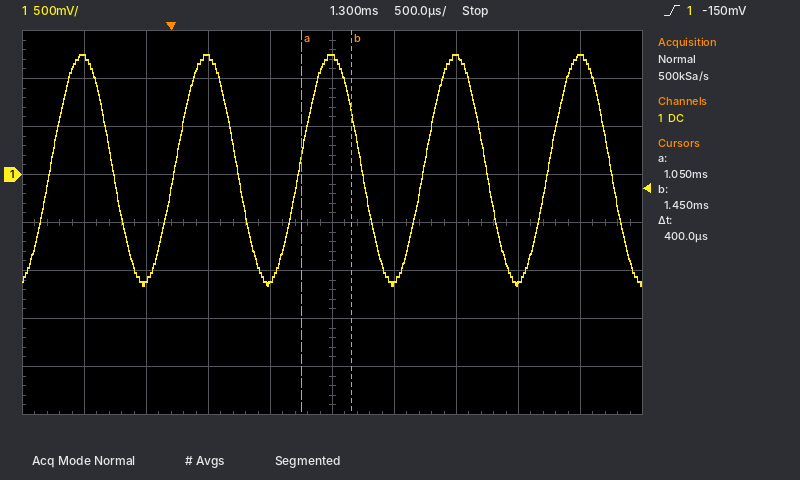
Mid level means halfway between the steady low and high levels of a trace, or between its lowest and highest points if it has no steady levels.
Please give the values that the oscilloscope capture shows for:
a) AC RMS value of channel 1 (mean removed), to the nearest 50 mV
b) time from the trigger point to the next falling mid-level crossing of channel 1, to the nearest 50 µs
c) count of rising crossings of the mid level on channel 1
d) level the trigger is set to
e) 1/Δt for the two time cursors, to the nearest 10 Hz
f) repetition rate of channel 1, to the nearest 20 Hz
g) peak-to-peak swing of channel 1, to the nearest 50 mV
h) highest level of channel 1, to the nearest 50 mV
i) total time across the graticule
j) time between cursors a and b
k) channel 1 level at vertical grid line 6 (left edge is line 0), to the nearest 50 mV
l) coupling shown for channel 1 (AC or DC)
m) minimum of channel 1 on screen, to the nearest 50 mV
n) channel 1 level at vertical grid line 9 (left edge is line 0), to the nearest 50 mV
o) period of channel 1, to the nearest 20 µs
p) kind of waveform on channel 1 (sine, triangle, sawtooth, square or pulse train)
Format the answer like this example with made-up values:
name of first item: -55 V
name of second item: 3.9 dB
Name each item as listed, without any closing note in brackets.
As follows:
AC RMS value of channel 1 (mean removed), to the nearest 50 mV: 850 mV
time from the trigger point to the next falling mid-level crossing of channel 1, to the nearest 50 µs: 550 µs
count of rising crossings of the mid level on channel 1: 5
level the trigger is set to: -150 mV
1/Δt for the two time cursors, to the nearest 10 Hz: 2.50 kHz
repetition rate of channel 1, to the nearest 20 Hz: 1.00 kHz
peak-to-peak swing of channel 1, to the nearest 50 mV: 2.40 V
highest level of channel 1, to the nearest 50 mV: 1.25 V
total time across the graticule: 5 ms
time between cursors a and b: 400 µs
channel 1 level at vertical grid line 6 (left edge is line 0), to the nearest 50 mV: -1.10 V
coupling shown for channel 1: DC
minimum of channel 1 on screen, to the nearest 50 mV: -1.15 V
channel 1 level at vertical grid line 9 (left edge is line 0), to the nearest 50 mV: 1.25 V
period of channel 1, to the nearest 20 µs: 1.00 ms
kind of waveform on channel 1: sine
